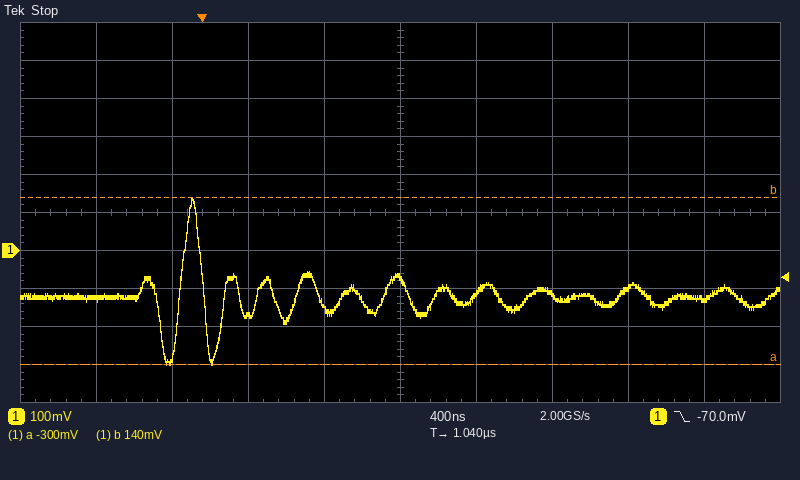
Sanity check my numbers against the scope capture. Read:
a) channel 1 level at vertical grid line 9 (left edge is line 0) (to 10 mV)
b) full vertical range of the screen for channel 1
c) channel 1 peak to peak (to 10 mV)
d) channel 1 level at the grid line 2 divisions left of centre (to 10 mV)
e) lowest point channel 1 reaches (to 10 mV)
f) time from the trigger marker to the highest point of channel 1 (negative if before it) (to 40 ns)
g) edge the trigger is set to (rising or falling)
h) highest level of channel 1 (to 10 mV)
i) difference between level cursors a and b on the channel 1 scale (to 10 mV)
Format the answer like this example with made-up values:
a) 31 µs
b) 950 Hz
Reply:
a) -130 mV
b) 1 V
c) 440 mV
d) -170 mV
e) -300 mV
f) -40 ns
g) falling
h) 140 mV
i) 440 mV
